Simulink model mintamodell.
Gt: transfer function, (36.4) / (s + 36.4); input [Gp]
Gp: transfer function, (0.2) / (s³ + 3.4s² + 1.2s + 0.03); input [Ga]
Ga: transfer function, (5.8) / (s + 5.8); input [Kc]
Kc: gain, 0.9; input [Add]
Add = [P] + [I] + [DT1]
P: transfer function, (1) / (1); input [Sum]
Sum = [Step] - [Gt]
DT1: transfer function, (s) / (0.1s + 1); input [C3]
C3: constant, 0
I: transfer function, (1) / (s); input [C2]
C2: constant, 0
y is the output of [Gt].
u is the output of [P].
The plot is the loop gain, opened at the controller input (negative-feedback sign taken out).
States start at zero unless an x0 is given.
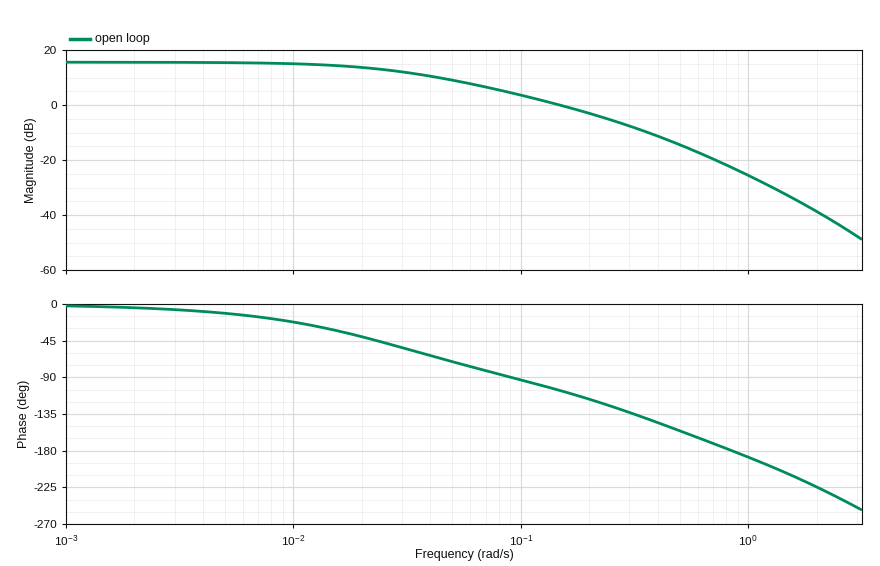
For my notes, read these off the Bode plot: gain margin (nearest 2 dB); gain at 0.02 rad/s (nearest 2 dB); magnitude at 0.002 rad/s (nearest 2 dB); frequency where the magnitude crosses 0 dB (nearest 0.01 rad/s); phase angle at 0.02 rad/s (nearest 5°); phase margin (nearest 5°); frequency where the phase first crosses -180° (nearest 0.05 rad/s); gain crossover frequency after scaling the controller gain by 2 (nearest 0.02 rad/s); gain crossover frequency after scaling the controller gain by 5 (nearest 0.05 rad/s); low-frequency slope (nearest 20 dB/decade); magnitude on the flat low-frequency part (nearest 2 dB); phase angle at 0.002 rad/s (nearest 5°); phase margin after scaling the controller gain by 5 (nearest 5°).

22 dB
14 dB
16 dB
0.15 rad/s
-40°
75°
0.85 rad/s
0.26 rad/s
0.50 rad/s
0 dB/decade
16 dB
-5°
25°
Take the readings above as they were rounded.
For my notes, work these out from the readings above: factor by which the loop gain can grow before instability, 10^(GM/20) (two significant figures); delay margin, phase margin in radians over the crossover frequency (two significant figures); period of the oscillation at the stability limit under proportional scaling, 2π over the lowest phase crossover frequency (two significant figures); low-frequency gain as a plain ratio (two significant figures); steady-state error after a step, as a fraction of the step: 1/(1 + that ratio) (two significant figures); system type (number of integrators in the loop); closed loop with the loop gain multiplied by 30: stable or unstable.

13
8.7 s
7.4 s
6.3
0.14
0
unstable
